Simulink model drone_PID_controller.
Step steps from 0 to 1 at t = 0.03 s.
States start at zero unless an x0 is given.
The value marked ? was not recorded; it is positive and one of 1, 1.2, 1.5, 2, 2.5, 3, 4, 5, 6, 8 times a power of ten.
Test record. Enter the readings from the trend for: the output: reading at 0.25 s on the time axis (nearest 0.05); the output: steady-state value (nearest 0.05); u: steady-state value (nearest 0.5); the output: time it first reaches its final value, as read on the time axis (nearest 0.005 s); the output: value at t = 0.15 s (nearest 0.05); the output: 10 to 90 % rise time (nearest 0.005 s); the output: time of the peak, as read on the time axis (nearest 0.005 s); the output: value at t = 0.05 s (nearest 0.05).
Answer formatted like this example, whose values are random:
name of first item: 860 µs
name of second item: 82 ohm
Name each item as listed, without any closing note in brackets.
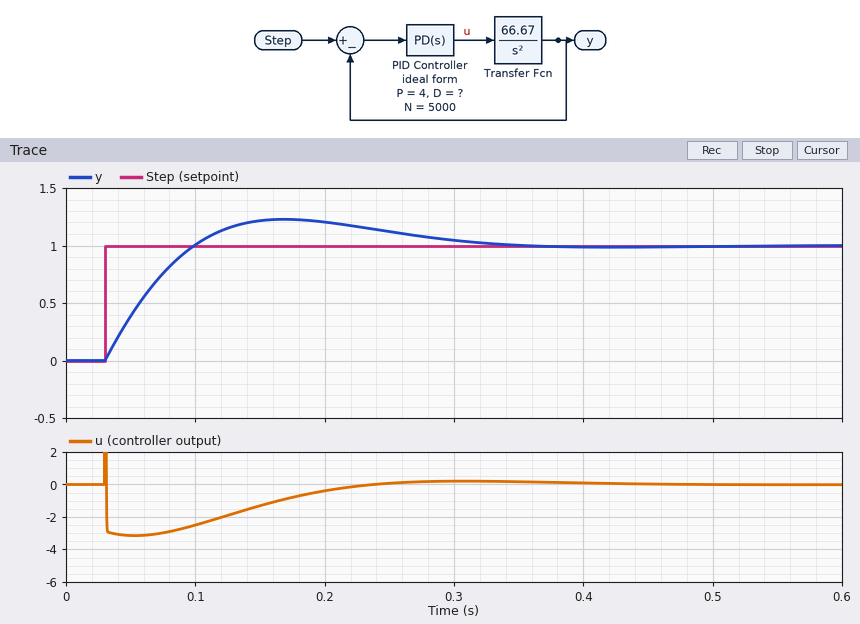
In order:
the output: reading at 0.25 s on the time axis: 1.10
the output: steady-state value: 1.00
u: steady-state value: 0.0
the output: time it first reaches its final value, as read on the time axis: 0.100 s
the output: value at t = 0.15 s: 1.20
the output: 10 to 90 % rise time: 0.055 s
the output: time of the peak, as read on the time axis: 0.170 s
the output: value at t = 0.05 s: 0.40
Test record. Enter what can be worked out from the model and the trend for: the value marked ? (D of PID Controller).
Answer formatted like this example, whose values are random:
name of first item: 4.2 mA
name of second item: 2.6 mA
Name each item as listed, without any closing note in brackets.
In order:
the value marked ?: 0.08
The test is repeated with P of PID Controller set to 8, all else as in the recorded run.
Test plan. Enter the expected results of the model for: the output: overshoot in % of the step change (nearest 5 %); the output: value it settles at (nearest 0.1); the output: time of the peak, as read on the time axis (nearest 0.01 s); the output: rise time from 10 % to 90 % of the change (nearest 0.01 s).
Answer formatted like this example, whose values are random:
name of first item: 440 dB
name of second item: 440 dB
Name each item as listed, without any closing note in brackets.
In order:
the output: overshoot in % of the step change: 15 %
the output: value it settles at: 1.0
the output: time of the peak, as read on the time axis: 0.12 s
the output: rise time from 10 % to 90 % of the change: 0.03 s
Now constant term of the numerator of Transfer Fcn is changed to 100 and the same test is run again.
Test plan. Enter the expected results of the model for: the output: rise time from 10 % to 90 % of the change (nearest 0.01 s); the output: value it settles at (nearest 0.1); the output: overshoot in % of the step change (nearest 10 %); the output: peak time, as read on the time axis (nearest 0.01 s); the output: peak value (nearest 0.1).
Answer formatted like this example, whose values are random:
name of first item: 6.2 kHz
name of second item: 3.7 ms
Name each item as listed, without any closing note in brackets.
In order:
the output: rise time from 10 % to 90 % of the change: 0.04 s
the output: value it settles at: 1.0
the output: overshoot in % of the step change: 20 %
the output: peak time, as read on the time axis: 0.14 s
the output: peak value: 1.2
